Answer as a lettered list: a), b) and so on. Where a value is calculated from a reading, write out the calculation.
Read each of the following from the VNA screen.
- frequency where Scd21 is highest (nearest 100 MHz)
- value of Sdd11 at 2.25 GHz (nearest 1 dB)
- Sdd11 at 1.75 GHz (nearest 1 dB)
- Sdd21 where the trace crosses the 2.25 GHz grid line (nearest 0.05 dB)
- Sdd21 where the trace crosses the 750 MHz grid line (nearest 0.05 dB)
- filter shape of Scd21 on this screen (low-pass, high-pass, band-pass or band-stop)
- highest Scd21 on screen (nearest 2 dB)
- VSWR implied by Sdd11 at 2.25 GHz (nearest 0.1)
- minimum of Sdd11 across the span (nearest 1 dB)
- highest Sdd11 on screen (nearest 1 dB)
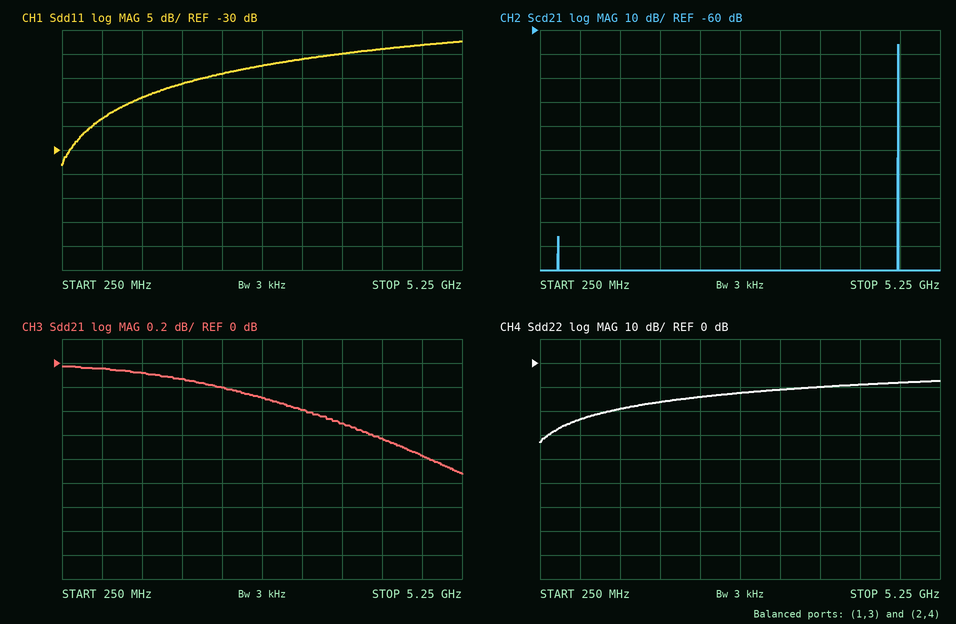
a) 4.7 GHz
b) -14 dB
c) -16 dB
d) -0.20 dB
e) -0.05 dB
f) band-pass
g) -66 dB
h) |Γ| = 10^(-14/20) = 0.1995; VSWR = (1 + 0.1995)/(1 − 0.1995) ≈ 1.5
i) -33 dB
j) -7 dB
